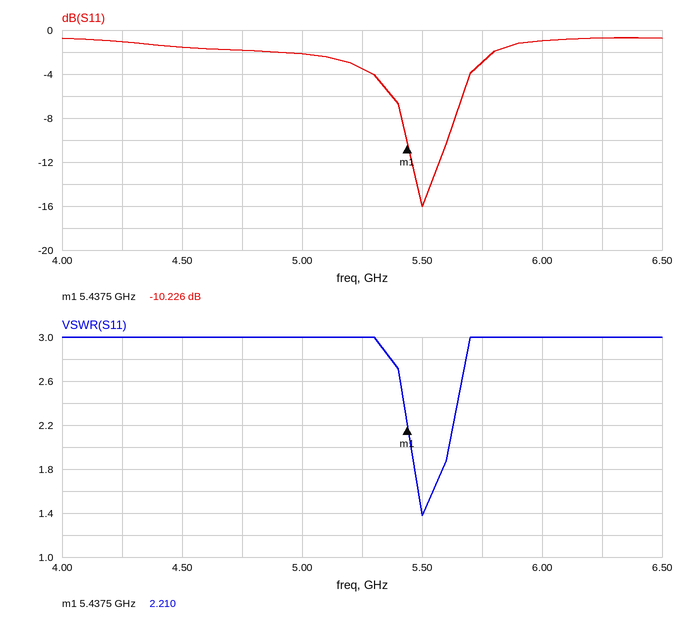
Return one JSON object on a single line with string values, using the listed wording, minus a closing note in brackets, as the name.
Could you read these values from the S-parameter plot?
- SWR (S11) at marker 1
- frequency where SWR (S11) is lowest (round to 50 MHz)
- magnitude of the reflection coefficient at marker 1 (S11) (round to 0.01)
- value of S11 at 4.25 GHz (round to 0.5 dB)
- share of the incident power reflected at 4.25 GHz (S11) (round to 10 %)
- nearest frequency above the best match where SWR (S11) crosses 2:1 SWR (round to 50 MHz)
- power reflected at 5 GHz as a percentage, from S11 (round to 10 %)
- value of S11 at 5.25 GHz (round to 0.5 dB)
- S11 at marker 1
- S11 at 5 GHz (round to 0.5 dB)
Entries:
{"SWR (S11) at marker 1": "2.210", "frequency where SWR (S11) is lowest": "5.50 GHz", "magnitude of the reflection coefficient at marker 1 (S11)": "0.31", "value of S11 at 4.25 GHz": "-1.0 dB", "share of the incident power reflected at 4.25 GHz (S11)": "80 %", "nearest frequency above the best match where SWR (S11) crosses 2:1 SWR": "5.60 GHz", "power reflected at 5 GHz as a percentage, from S11": "60 %", "value of S11 at 5.25 GHz": "-3.5 dB", "S11 at marker 1": "-10.226 dB", "S11 at 5 GHz": "-2.0 dB"}
